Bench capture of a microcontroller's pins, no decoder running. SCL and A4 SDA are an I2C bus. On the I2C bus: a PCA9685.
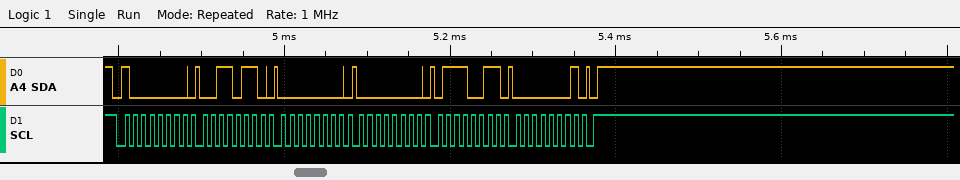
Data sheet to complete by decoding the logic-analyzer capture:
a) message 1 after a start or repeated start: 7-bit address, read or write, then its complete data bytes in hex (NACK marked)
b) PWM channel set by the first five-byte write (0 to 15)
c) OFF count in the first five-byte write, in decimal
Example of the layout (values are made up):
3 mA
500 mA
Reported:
0x40 write: 36 00 00 73 01
12
371
